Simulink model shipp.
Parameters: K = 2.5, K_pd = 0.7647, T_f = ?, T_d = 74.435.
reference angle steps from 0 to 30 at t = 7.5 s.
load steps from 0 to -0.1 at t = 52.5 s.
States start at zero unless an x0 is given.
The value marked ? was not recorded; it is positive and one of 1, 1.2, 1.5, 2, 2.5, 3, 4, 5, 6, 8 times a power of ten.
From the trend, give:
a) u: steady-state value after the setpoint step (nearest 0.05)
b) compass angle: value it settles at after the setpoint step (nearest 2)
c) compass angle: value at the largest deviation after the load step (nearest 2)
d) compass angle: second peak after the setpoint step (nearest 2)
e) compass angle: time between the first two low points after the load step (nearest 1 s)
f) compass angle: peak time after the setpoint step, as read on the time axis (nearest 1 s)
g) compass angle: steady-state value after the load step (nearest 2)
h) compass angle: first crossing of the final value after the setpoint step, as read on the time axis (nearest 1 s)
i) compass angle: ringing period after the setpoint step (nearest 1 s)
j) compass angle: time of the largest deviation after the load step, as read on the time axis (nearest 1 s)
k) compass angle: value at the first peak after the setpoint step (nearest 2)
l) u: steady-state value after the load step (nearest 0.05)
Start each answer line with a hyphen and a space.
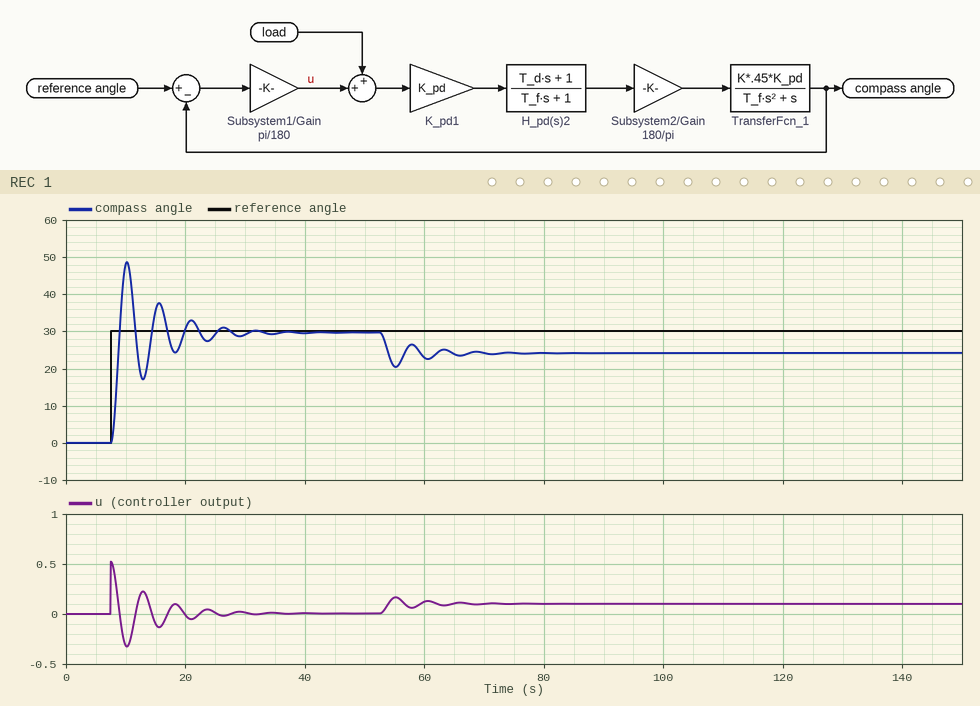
- 0.00
- 30
- 20
- 38
- 5 s
- 10 s
- 24
- 9 s
- 5 s
- 55 s
- 48
- 0.10
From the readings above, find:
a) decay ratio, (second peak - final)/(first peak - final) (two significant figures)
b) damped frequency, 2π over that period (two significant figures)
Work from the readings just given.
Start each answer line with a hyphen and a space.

- 0.44
- 1.3 rad/s
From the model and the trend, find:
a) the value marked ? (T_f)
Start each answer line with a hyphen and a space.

- 6
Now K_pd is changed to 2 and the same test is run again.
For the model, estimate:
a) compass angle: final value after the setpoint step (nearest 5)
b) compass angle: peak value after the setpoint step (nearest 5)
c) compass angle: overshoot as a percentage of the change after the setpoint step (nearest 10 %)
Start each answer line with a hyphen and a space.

- 30
- 55
- 80 %
